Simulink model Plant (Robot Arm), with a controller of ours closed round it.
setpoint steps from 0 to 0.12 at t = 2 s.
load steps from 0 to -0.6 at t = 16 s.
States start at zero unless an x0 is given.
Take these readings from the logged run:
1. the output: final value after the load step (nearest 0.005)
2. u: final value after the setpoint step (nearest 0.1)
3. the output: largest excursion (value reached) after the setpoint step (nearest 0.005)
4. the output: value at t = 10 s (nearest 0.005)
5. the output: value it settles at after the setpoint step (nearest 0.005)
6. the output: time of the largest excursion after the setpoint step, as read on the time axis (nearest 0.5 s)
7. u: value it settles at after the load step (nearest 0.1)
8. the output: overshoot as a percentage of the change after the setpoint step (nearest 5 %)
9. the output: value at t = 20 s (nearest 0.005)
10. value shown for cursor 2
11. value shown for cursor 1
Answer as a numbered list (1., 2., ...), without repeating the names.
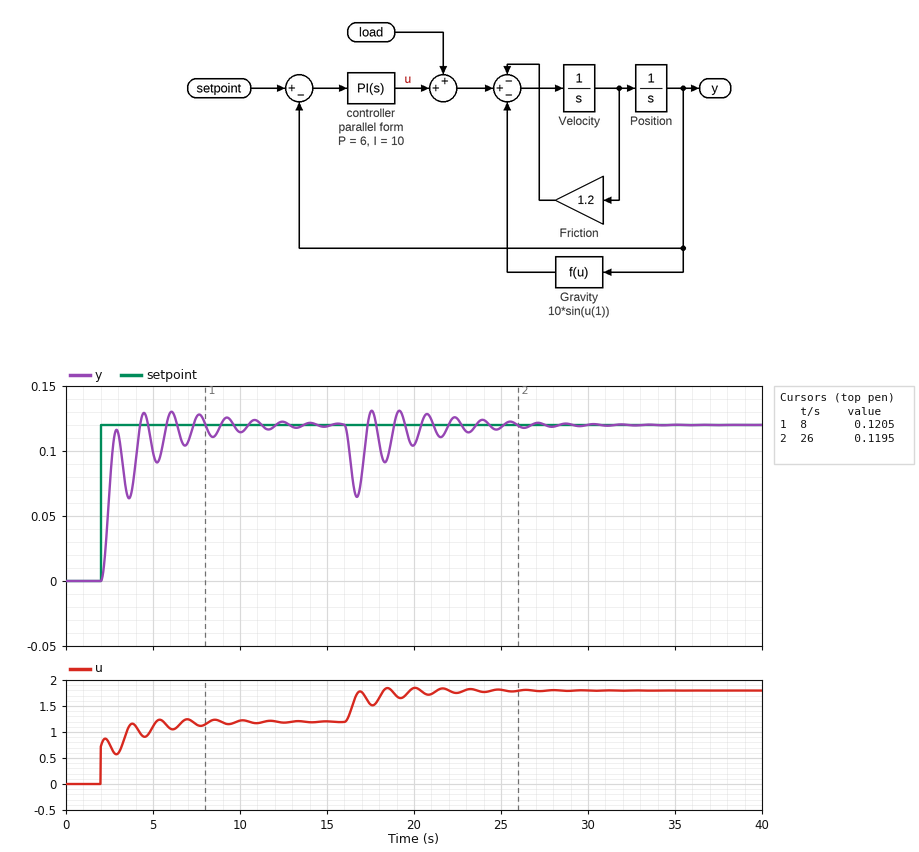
1. 0.120
2. 1.2
3. 0.130
4. 0.115
5. 0.120
6. 6.0 s
7. 1.8
8. 10 %
9. 0.105
10. 0.1195
11. 0.1205
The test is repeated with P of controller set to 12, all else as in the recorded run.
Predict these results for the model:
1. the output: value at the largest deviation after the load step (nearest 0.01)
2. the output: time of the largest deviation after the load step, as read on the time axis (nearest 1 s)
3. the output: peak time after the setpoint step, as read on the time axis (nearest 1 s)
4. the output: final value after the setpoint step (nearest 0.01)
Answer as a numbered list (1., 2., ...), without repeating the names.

1. 0.08
2. 17 s
3. 3 s
4. 0.12
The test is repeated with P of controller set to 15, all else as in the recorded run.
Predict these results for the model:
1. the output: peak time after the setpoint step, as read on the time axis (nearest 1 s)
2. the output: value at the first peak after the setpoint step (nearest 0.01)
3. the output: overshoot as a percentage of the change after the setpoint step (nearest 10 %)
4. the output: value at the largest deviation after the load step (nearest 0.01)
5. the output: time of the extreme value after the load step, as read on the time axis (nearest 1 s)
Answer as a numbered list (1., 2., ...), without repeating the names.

1. 3 s
2. 0.14
3. 20 %
4. 0.08
5. 17 s
